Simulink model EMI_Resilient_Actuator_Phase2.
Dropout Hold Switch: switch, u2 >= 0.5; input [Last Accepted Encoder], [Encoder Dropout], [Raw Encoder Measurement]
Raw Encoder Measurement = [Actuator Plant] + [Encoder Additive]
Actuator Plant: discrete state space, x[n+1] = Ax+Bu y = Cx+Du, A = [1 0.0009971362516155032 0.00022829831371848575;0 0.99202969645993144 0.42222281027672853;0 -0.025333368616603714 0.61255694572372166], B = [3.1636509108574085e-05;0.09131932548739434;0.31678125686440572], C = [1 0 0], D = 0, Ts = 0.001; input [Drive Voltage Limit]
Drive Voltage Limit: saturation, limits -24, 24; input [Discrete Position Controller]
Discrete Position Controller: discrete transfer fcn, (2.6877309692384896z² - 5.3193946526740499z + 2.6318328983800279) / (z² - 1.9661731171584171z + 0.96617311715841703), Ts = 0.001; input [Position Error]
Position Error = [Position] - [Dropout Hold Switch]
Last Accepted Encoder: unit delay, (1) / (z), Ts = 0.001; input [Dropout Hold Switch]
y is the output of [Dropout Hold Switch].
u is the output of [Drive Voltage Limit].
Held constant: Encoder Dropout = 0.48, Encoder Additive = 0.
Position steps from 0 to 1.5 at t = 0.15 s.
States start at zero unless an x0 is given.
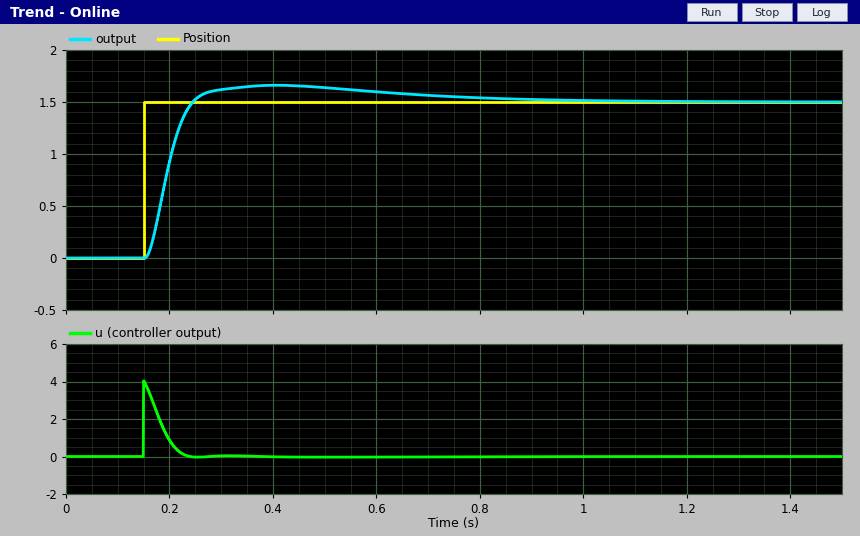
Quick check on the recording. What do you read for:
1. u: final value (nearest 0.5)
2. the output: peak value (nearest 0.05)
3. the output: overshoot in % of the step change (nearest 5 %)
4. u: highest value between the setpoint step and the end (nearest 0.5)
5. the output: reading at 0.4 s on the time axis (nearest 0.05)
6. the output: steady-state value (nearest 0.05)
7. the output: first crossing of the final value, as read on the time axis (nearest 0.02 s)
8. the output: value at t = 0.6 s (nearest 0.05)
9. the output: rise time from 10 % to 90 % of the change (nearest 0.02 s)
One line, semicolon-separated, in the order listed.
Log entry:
0.0; 1.65; 10 %; 4.0; 1.65; 1.50; 0.24 s; 1.60; 0.06 s
